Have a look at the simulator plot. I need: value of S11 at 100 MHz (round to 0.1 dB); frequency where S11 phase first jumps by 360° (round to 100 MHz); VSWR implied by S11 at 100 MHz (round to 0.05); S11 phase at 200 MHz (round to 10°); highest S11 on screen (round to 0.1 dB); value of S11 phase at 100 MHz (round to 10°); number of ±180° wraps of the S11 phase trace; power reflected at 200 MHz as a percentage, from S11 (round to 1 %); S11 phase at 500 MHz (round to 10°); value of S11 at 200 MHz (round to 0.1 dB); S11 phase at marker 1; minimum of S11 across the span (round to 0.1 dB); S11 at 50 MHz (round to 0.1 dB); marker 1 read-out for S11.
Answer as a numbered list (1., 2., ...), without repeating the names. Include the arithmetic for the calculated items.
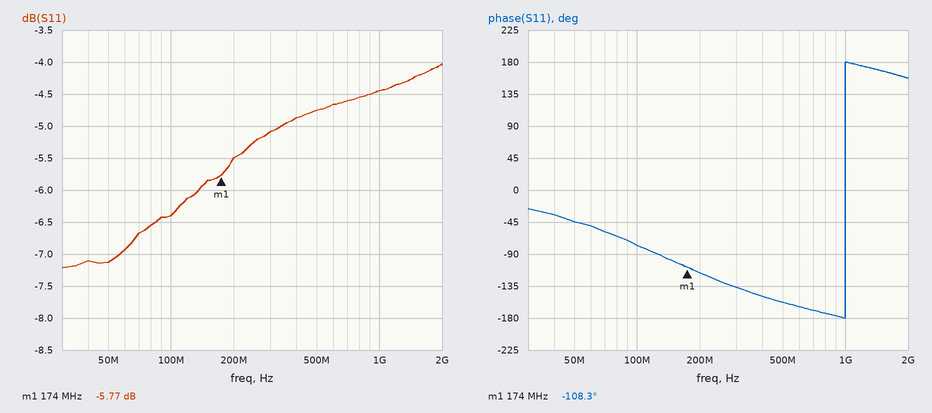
1. -6.4 dB
2. 1.0 GHz
3. |Γ| = 10^(-6.4/20) = 0.4786; VSWR = (1 + 0.4786)/(1 − 0.4786) ≈ 2.84, so 2.85 to the nearest 0.05
4. -120°
5. -4.0 dB
6. -80°
7. 1
8. 10^(-5.5/10) ≈ 28 %
9. -160°
10. -5.5 dB
11. -108.3°
12. -7.2 dB
13. -7.1 dB
14. -5.77 dB
